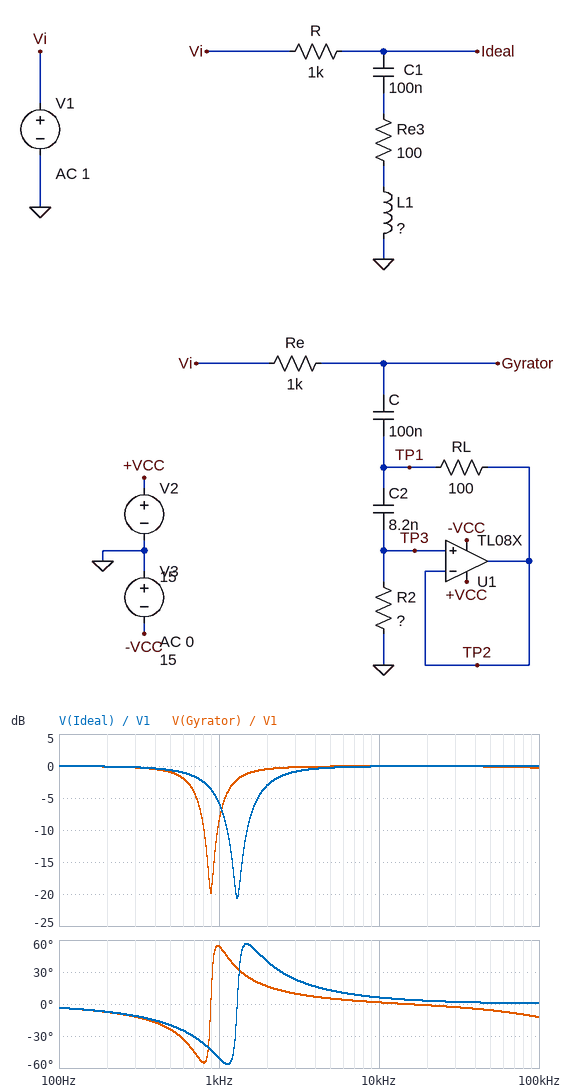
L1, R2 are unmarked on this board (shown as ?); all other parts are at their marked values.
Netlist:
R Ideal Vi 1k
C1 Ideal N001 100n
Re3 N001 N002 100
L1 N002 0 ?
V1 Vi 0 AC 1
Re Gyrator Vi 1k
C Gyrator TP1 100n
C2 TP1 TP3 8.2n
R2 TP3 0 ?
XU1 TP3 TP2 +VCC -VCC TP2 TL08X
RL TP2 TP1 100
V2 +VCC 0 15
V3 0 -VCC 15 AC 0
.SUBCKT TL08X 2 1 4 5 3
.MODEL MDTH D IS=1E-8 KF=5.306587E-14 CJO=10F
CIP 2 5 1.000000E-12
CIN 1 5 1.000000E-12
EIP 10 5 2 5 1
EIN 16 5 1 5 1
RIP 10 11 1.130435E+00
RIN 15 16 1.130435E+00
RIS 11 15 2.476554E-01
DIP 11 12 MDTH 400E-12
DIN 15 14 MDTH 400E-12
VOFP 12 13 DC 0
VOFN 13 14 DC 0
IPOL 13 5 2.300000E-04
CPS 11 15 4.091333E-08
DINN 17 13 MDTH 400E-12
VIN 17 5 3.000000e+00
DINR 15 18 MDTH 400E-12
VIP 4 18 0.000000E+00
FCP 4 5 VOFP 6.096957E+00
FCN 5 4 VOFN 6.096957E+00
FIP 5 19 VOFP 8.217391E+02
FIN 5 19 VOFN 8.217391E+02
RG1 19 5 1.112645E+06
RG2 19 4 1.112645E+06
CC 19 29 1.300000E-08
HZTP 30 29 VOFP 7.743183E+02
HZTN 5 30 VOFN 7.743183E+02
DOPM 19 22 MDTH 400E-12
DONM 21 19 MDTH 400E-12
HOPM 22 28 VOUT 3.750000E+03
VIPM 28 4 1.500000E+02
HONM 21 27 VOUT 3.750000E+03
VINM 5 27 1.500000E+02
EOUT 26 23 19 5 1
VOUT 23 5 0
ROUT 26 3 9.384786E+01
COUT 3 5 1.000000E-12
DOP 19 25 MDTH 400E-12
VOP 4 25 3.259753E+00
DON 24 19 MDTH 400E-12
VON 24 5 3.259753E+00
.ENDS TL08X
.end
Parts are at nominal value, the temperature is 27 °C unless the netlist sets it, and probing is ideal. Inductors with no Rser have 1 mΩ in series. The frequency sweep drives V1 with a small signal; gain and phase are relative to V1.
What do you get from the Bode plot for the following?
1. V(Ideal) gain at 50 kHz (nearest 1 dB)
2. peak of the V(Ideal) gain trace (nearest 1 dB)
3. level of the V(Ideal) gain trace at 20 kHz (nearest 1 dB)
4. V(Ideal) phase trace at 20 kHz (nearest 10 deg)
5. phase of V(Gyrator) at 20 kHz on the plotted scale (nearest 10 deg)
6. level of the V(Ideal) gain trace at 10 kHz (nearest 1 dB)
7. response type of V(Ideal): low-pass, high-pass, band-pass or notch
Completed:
0 dB
0 dB
0 dB
0 deg
0 deg
0 dB
notch
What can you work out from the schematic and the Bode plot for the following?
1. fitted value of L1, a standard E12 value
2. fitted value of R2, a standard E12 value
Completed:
150 mH
390 kΩ
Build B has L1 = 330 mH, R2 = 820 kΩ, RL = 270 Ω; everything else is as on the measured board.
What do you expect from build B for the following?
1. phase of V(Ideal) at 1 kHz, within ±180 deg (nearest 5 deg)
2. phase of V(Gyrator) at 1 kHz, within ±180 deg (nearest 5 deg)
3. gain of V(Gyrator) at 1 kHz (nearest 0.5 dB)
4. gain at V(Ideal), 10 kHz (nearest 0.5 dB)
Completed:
55 deg
5 deg
0 dB
0 dB
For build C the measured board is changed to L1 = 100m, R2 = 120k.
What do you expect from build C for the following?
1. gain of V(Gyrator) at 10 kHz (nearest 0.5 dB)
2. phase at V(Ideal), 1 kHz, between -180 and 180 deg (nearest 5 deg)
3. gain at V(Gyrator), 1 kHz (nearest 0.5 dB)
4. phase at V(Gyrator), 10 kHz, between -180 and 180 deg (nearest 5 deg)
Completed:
0 dB
-45 deg
-3.5 dB
10 deg
